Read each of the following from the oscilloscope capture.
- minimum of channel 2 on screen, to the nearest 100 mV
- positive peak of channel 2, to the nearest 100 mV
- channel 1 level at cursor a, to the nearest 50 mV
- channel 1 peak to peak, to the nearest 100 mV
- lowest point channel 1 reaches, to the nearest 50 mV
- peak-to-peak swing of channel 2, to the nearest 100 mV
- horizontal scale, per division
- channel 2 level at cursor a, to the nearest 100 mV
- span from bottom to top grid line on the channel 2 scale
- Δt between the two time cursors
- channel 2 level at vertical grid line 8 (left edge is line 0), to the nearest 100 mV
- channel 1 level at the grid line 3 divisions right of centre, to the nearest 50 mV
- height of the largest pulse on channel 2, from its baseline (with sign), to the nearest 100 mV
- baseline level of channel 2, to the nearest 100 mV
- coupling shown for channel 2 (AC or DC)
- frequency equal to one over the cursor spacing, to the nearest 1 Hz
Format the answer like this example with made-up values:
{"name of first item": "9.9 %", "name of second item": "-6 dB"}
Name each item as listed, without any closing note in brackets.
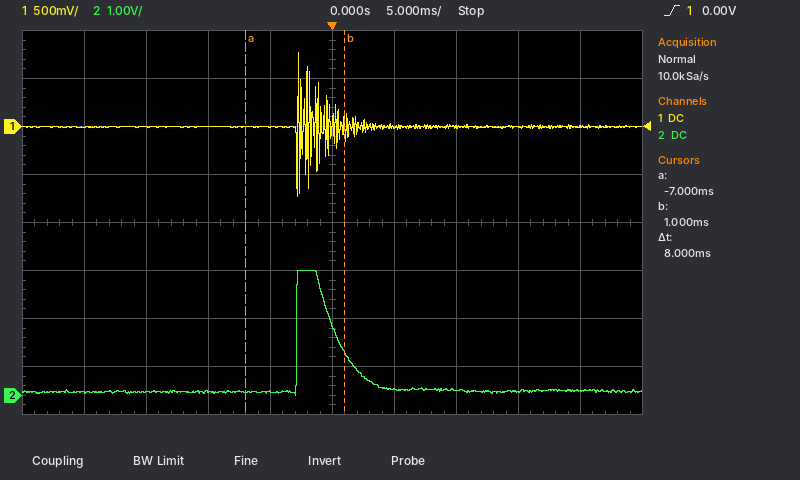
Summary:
{"minimum of channel 2 on screen, to the nearest 100 mV": "0.0 V", "positive peak of channel 2, to the nearest 100 mV": "2.6 V", "channel 1 level at cursor a, to the nearest 50 mV": "0 mV", "channel 1 peak to peak, to the nearest 100 mV": "1.50 V", "lowest point channel 1 reaches, to the nearest 50 mV": "-750 mV", "peak-to-peak swing of channel 2, to the nearest 100 mV": "2.6 V", "horizontal scale, per division": "5 ms", "channel 2 level at cursor a, to the nearest 100 mV": "100 mV", "span from bottom to top grid line on the channel 2 scale": "8 V", "Δt between the two time cursors": "8 ms", "channel 2 level at vertical grid line 8 (left edge is line 0), to the nearest 100 mV": "100 mV", "channel 1 level at the grid line 3 divisions right of centre, to the nearest 50 mV": "0 mV", "height of the largest pulse on channel 2, from its baseline (with sign), to the nearest 100 mV": "+2.5 V", "baseline level of channel 2, to the nearest 100 mV": "100 mV", "coupling shown for channel 2": "DC", "frequency equal to one over the cursor spacing, to the nearest 1 Hz": "125 Hz"}
